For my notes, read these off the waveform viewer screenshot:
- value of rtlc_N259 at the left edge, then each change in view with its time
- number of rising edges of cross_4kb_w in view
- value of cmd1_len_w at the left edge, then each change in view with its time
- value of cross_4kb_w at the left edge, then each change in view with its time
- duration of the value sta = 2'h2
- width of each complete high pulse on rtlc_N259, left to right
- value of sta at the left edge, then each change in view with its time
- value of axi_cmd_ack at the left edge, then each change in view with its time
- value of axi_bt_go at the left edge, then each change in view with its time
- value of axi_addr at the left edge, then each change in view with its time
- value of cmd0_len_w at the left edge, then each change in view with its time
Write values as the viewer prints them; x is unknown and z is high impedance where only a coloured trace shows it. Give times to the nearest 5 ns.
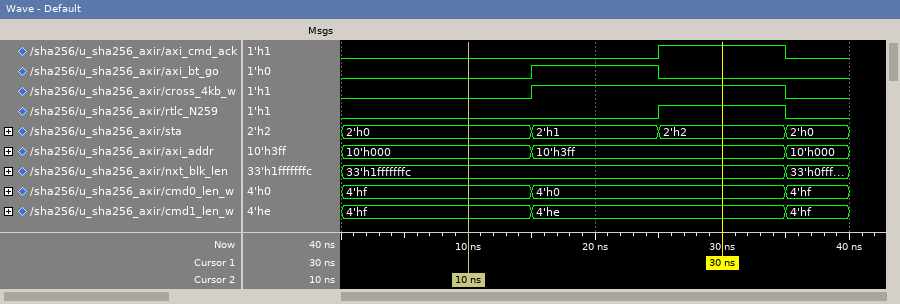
0, 1 at 25 ns, 0 at 35 ns
1
4'hf, 4'he at 15 ns, 4'hf at 35 ns
0, 1 at 15 ns, 0 at 35 ns
10 ns
10 ns
2'h0, 2'h1 at 15 ns, 2'h2 at 25 ns, 2'h0 at 35 ns
0, 1 at 25 ns, 0 at 35 ns
0, 1 at 15 ns, 0 at 25 ns
10'h000, 10'h3ff at 15 ns, 10'h000 at 35 ns
4'hf, 4'h0 at 15 ns, 4'hf at 35 ns
